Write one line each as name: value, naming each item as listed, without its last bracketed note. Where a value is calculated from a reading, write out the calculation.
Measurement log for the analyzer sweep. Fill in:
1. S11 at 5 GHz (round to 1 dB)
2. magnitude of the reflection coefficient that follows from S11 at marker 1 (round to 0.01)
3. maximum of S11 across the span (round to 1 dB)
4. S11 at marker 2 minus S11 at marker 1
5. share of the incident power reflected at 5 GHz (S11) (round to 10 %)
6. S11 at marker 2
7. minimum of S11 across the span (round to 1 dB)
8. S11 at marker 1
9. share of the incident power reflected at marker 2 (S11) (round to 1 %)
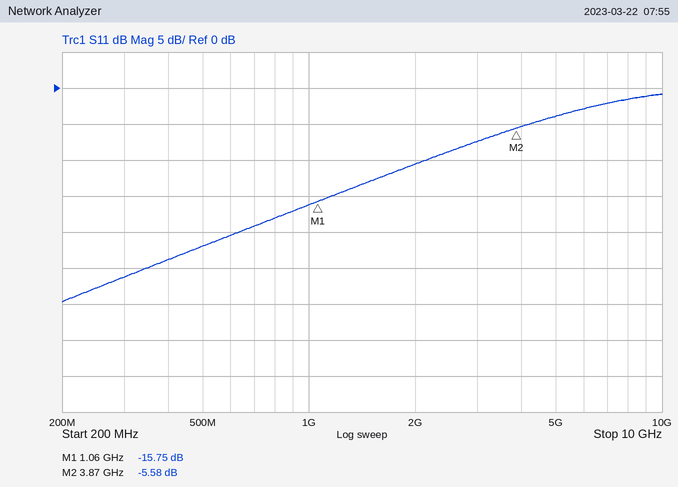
S11 at 5 GHz: -4 dB
magnitude of the reflection coefficient that follows from S11 at marker 1: 10^(-15.75/20) ≈ 0.16
maximum of S11 across the span: -1 dB
S11 at marker 2 minus S11 at marker 1: -5.58 − (-15.75) = 10.17 dB
share of the incident power reflected at 5 GHz (S11): 10^(-4/10) ≈ 40 %
S11 at marker 2: -5.58 dB
minimum of S11 across the span: -30 dB
S11 at marker 1: -15.75 dB
share of the incident power reflected at marker 2 (S11): 10^(-5.58/10) ≈ 28 %
